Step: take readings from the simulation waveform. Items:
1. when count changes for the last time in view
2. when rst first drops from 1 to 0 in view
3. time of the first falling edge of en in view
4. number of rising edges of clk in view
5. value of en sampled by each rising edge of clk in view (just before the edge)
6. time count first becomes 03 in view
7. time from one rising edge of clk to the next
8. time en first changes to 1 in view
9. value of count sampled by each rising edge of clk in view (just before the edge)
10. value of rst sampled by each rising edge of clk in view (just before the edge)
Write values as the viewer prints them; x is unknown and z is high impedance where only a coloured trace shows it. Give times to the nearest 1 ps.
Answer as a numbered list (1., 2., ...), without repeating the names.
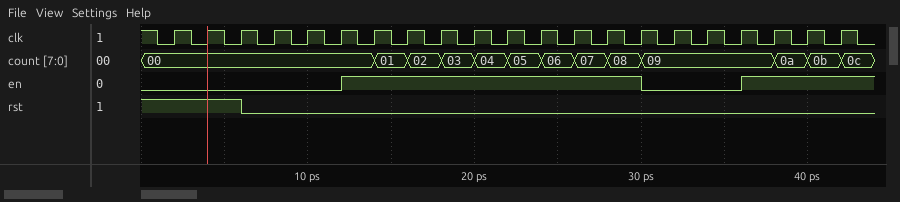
1. 42 ps
2. 6 ps
3. 30 ps
4. 21
5. 0 0 0 0 0 0 1 1 1 1 1 1 1 1 1 0 0 0 1 1 1
6. 18 ps
7. 2 ps
8. 12 ps
9. 00, 00, 00, 00, 00, 00, 00, 01, 02, 03, 04, 05, 06, 07, 08, 09, 09, 09, 09, 0a, 0b
10. 1 1 1 0 0 0 0 0 0 0 0 0 0 0 0 0 0 0 0 0 0
